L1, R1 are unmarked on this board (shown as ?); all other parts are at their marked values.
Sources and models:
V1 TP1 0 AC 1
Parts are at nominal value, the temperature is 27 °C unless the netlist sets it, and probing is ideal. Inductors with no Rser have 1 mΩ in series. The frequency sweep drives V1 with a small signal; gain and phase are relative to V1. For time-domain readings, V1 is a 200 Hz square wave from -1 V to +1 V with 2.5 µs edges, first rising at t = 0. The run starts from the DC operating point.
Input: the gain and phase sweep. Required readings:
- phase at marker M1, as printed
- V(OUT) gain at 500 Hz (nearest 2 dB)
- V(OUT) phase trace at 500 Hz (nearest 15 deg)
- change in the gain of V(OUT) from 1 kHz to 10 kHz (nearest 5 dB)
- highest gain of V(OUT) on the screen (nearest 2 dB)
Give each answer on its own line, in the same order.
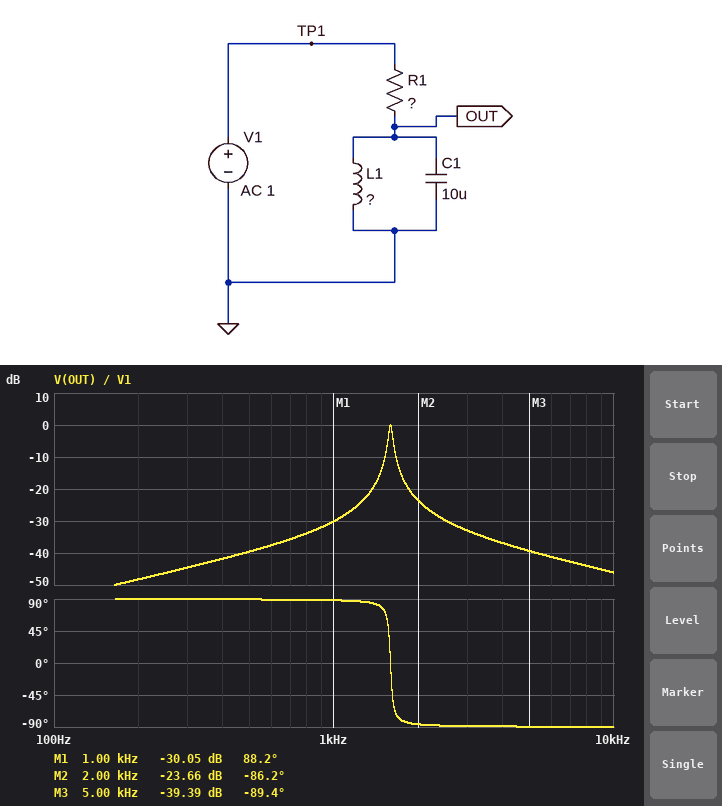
88.2 deg
-40 dB
90 deg
-15 dB
0 dB
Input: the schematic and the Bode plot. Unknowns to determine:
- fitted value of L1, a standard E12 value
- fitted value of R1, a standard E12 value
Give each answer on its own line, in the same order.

1 mH
330 Ω
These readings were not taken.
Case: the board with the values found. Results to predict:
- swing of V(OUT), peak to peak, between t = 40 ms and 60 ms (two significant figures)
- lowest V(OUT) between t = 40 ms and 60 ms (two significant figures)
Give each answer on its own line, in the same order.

71 mV
-35 mV
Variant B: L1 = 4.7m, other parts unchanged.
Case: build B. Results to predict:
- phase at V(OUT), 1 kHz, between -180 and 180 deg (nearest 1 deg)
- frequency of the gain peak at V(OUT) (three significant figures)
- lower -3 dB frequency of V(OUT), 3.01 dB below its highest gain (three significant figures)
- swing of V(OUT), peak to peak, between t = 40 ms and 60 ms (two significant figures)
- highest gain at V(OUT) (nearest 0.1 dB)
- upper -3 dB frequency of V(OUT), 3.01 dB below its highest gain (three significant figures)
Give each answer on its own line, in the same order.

-84 deg
734 Hz
710 Hz
170 mV
0 dB
759 Hz
